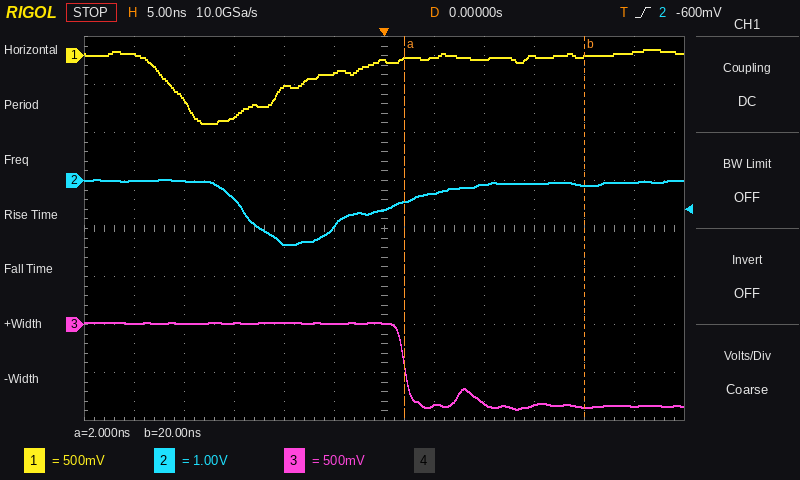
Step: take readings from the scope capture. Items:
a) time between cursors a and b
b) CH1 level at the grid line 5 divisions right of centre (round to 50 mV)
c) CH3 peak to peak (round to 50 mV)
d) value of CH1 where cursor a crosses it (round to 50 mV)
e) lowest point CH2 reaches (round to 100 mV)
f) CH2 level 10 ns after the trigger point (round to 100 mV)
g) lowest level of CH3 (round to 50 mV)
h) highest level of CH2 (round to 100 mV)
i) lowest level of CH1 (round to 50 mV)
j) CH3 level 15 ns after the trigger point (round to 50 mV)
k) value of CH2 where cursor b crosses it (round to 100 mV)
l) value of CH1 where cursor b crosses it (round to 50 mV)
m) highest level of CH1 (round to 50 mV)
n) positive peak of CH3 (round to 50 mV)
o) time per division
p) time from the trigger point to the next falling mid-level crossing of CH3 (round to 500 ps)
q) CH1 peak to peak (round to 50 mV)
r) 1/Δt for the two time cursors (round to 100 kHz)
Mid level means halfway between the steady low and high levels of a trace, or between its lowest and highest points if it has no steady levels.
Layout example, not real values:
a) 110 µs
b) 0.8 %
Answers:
a) 18.0 ns
b) 50 mV
c) 900 mV
d) -50 mV
e) -1.3 V
f) -100 mV
g) -900 mV
h) 0.0 V
i) -700 mV
j) -850 mV
k) -100 mV
l) 0 mV
m) 50 mV
n) 0 mV
o) 5 ns
p) 2.0 ns
q) 750 mV
r) 55.6 MHz
